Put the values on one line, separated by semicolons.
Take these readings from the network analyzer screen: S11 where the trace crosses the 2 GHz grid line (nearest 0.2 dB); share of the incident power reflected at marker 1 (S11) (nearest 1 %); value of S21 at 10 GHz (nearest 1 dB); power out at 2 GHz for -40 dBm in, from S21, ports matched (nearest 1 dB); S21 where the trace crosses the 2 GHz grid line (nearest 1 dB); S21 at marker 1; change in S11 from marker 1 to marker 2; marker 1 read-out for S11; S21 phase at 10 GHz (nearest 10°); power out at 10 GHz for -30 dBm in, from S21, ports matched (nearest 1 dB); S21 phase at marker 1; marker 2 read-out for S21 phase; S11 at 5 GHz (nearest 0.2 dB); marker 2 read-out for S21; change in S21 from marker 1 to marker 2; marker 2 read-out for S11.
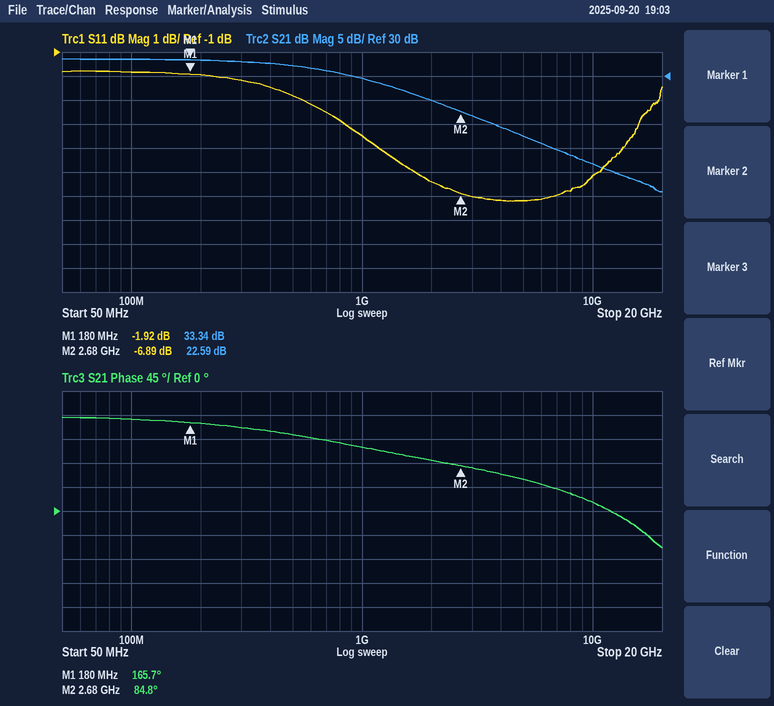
-6.4 dB; 64 %; 12 dB; -15 dBm; 25 dB; 33.34 dB; -4.97 dB; -1.92 dB; 20°; -18 dBm; 165.7°; 84.8°; -7.2 dB; 22.59 dB; -10.75 dB; -6.89 dB
